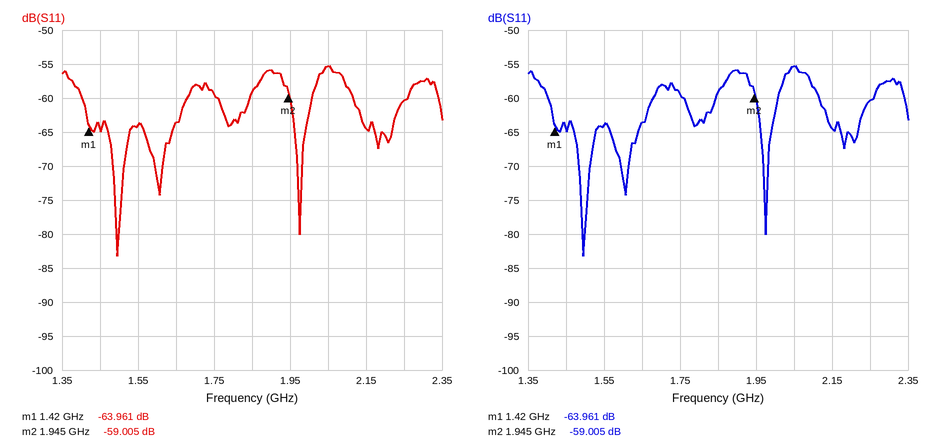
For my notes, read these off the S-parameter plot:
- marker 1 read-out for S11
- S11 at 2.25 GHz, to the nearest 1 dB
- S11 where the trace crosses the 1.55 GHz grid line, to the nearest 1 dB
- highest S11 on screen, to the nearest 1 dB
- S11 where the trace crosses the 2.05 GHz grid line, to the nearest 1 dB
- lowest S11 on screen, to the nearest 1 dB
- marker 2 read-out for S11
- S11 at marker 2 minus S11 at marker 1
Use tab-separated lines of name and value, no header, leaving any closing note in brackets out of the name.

marker 1 read-out for S11	-63.961 dB
S11 at 2.25 GHz, to the nearest 1 dB	-60 dB
S11 where the trace crosses the 1.55 GHz grid line, to the nearest 1 dB	-64 dB
highest S11 on screen, to the nearest 1 dB	-55 dB
S11 where the trace crosses the 2.05 GHz grid line, to the nearest 1 dB	-55 dB
lowest S11 on screen, to the nearest 1 dB	-83 dB
marker 2 read-out for S11	-59.005 dB
S11 at marker 2 minus S11 at marker 1	4.956 dB
